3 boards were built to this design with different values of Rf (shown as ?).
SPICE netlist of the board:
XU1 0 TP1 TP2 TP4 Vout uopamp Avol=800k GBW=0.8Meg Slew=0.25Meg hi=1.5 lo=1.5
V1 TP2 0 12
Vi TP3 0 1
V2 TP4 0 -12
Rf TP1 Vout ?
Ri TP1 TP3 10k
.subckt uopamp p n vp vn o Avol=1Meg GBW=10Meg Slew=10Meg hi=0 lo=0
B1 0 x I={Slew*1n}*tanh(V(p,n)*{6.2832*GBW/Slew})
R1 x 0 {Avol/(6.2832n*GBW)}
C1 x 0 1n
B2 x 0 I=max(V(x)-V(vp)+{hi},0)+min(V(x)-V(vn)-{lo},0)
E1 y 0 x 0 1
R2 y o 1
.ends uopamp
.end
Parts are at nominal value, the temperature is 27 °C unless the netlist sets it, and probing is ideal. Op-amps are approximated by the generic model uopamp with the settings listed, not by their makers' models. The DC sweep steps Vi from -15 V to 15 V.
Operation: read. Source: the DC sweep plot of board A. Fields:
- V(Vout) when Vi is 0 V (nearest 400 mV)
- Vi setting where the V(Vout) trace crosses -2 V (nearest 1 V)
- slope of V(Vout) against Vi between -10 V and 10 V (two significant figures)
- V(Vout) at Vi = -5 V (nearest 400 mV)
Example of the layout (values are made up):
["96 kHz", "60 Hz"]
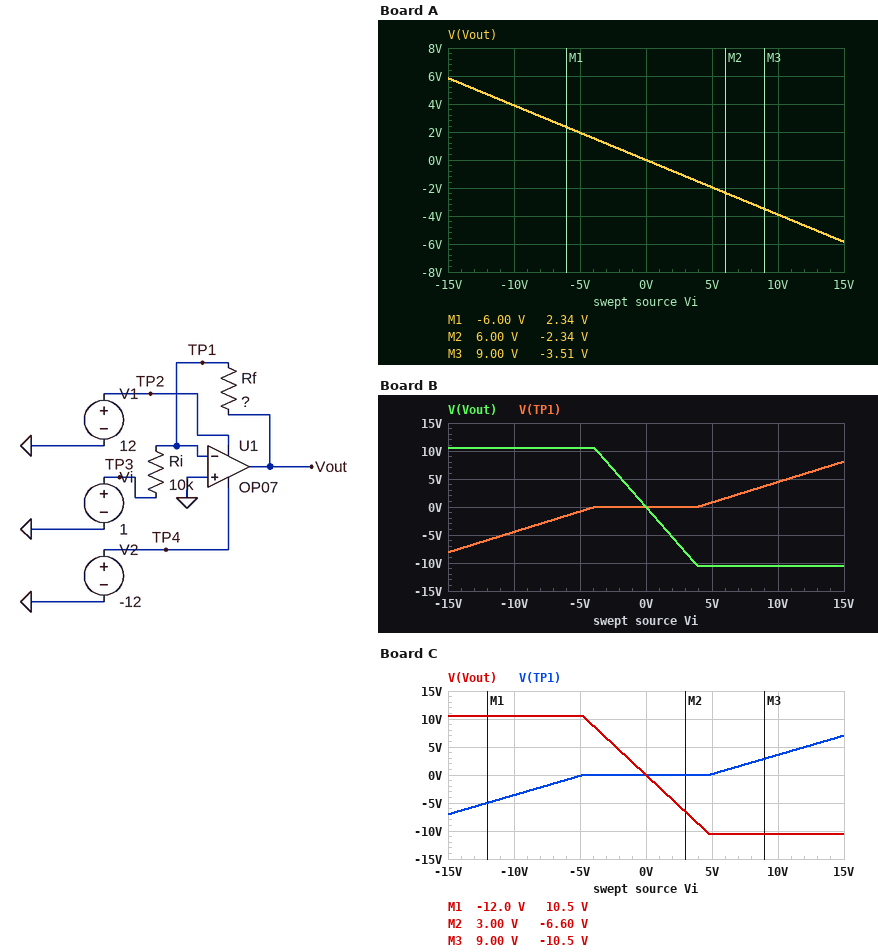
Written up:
["0 V", "5 V", "-0.39 V/V", "2.0 V"]
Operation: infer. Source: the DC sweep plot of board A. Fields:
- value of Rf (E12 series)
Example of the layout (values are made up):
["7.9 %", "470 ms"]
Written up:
["3.9 kΩ"]
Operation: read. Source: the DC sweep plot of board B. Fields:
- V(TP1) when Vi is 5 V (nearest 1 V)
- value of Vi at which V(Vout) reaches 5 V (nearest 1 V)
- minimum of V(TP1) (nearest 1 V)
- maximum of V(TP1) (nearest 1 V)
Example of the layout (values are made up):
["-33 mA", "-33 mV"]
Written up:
["1 V", "-2 V", "-8 V", "8 V"]
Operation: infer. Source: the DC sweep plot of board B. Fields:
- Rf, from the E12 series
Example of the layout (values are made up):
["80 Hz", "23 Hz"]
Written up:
["27 kΩ"]
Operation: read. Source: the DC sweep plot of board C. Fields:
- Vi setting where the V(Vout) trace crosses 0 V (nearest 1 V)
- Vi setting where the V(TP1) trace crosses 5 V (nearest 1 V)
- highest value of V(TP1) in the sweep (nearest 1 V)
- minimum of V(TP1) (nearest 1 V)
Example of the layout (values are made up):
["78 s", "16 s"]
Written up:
["0 V", "12 V", "7 V", "-7 V"]
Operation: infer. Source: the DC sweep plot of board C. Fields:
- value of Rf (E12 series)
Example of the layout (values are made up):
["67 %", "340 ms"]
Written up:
["22 kΩ"]
